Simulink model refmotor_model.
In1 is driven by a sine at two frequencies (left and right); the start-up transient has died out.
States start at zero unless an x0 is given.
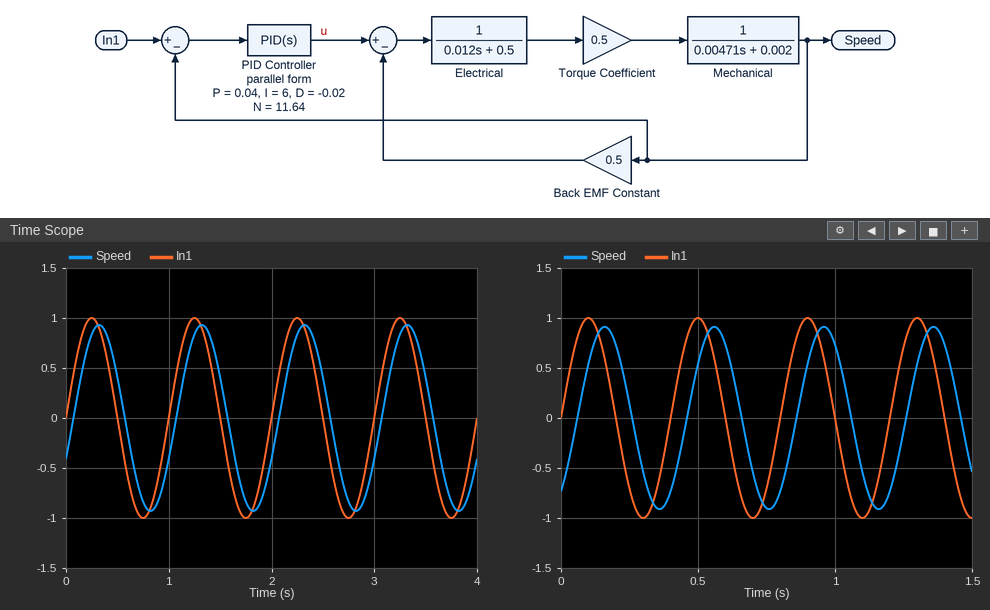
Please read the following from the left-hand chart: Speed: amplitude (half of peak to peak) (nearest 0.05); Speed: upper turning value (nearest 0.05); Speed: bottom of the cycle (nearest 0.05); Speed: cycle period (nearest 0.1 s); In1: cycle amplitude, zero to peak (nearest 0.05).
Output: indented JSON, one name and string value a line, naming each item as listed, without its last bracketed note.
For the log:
{
  "Speed: amplitude (half of peak to peak)": "0.95",
  "Speed: upper turning value": "0.95",
  "Speed: bottom of the cycle": "-0.95",
  "Speed: cycle period": "1.0 s",
  "In1: cycle amplitude, zero to peak": "1.00"
}
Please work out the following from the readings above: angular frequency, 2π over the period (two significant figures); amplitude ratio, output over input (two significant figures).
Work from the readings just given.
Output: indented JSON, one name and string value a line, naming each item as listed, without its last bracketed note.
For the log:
{
  "angular frequency, 2π over the period": "6.3 rad/s",
  "amplitude ratio, output over input": "0.95"
}
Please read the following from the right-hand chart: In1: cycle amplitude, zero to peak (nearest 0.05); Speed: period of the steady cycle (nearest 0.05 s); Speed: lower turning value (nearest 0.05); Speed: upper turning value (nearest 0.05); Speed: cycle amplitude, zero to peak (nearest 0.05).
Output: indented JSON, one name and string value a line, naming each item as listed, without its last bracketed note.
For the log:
{
  "In1: cycle amplitude, zero to peak": "1.00",
  "Speed: period of the steady cycle": "0.40 s",
  "Speed: lower turning value": "-0.90",
  "Speed: upper turning value": "0.90",
  "Speed: cycle amplitude, zero to peak": "0.90"
}
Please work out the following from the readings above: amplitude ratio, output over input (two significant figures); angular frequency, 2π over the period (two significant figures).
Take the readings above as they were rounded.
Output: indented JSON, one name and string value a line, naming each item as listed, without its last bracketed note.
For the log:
{
  "amplitude ratio, output over input": "0.90",
  "angular frequency, 2π over the period": "16 rad/s"
}
